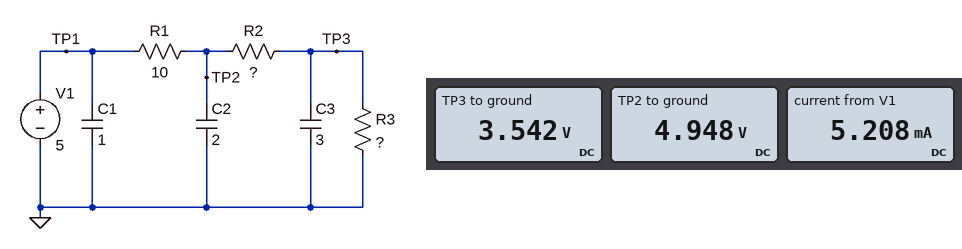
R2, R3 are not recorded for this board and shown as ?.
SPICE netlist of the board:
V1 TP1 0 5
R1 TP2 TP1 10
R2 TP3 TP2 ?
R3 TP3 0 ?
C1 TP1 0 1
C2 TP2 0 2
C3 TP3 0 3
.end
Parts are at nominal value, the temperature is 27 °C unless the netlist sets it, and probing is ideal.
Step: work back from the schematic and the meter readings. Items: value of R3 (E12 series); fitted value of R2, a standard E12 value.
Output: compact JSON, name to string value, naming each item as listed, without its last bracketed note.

{"value of R3": "680 Ω", "fitted value of R2, a standard E12 value": "270 Ω"}
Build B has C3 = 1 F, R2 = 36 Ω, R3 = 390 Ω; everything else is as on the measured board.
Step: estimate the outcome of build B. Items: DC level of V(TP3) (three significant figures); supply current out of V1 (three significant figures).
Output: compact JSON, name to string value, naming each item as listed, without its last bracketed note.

{"DC level of V(TP3)": "4.47 V", "supply current out of V1": "11.5 mA"}
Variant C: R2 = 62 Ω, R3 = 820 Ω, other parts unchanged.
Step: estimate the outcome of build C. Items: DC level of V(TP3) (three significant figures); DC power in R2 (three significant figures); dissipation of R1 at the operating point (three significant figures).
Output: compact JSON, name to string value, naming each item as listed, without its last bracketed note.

{"DC level of V(TP3)": "4.60 V", "DC power in R2": "1.95 mW", "dissipation of R1 at the operating point": "314 µW"}
